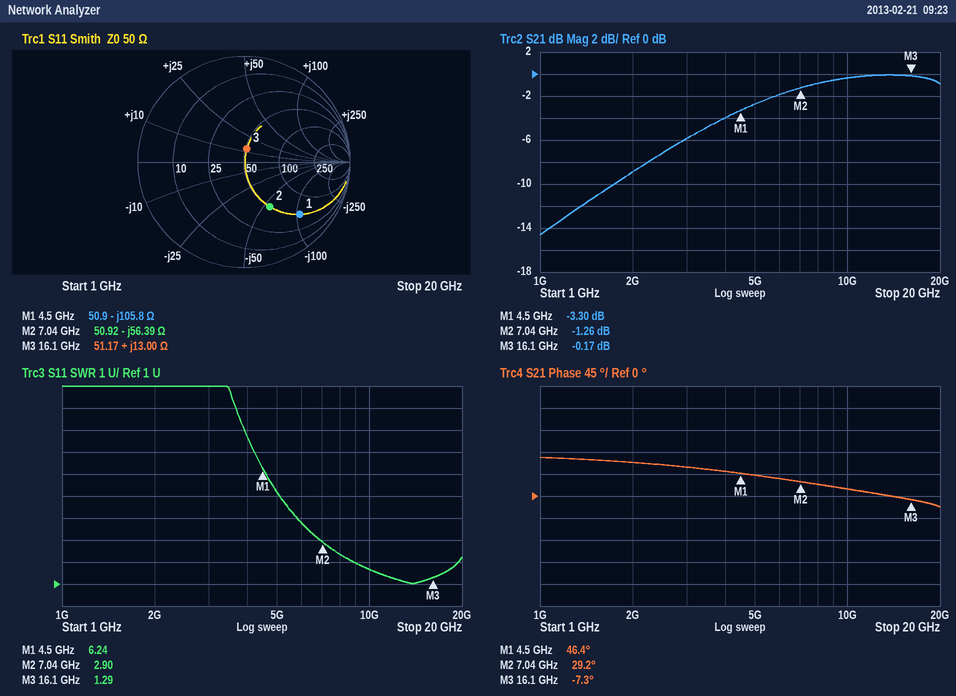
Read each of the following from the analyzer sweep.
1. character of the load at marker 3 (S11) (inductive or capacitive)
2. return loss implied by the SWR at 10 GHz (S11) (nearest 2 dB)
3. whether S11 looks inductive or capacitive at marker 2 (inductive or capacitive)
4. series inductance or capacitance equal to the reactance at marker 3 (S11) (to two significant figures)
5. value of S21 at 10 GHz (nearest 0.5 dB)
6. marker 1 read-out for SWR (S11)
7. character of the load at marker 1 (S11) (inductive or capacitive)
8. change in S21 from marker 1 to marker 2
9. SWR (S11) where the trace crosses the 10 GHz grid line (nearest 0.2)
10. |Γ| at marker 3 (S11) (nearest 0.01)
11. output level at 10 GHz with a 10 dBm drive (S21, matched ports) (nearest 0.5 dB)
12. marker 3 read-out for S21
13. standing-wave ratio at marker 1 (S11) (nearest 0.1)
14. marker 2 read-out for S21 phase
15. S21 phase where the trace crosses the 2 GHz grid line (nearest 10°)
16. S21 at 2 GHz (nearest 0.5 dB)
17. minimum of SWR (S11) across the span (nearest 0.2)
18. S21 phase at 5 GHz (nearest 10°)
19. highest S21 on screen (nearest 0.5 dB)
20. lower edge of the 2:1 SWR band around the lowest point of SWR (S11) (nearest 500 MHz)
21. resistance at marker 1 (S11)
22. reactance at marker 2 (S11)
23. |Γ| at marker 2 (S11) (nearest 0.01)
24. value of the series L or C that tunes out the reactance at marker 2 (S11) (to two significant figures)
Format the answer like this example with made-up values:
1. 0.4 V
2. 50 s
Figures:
1. inductive
2. 12 dB
3. capacitive
4. 130 pH
5. -0.5 dB
6. 6.24
7. capacitive
8. 2.04 dB
9. 1.6
10. 0.13
11. 9.5 dBm
12. -0.17 dB
13. 6.2
14. 29.2°
15. 70°
16. -9.0 dB
17. 1.0
18. 40°
19. 0.0 dB
20. 9.0 GHz
21. 50.9 Ω
22. -56.39 Ω
23. 0.49
24. 1.3 nH
